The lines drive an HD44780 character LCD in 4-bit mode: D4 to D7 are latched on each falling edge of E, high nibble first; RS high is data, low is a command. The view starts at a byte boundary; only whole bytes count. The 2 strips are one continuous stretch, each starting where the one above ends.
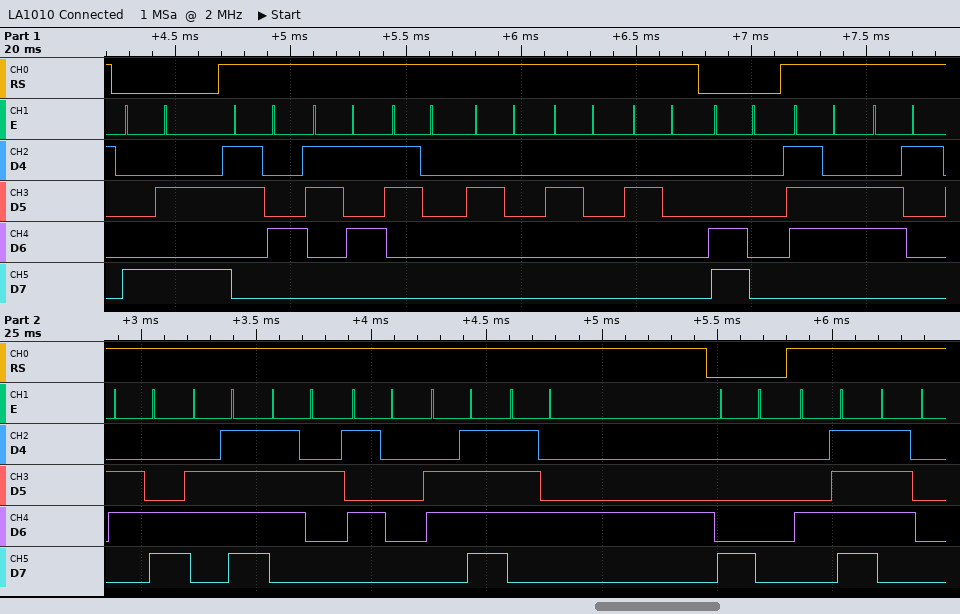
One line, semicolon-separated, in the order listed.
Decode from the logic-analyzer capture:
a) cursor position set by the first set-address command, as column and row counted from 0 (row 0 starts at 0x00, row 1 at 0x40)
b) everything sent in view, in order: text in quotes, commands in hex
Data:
column 10, row 0; 0x8A "450   " 0xC0 "valorPot" 0x80 "Op"
